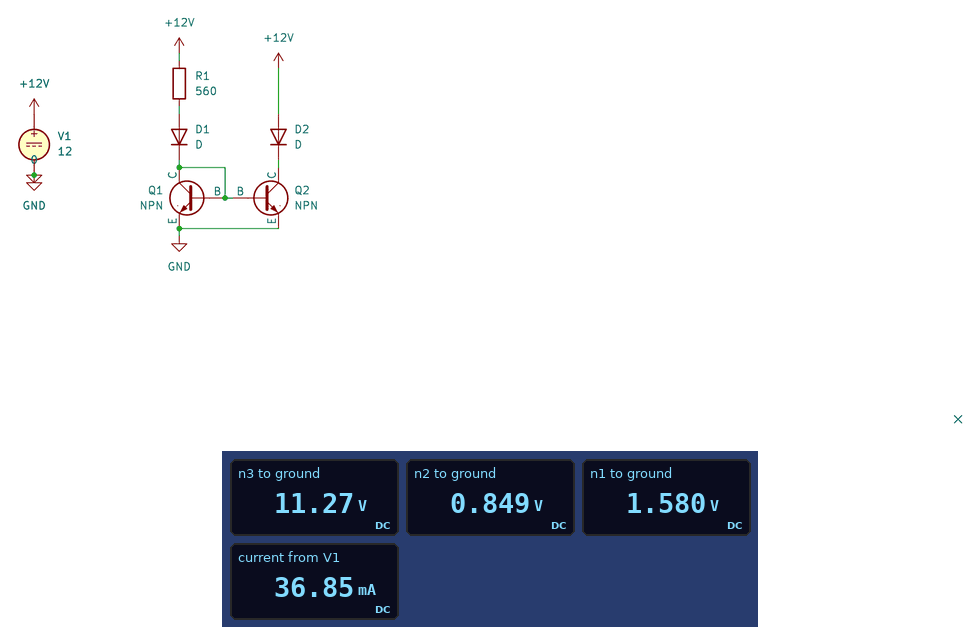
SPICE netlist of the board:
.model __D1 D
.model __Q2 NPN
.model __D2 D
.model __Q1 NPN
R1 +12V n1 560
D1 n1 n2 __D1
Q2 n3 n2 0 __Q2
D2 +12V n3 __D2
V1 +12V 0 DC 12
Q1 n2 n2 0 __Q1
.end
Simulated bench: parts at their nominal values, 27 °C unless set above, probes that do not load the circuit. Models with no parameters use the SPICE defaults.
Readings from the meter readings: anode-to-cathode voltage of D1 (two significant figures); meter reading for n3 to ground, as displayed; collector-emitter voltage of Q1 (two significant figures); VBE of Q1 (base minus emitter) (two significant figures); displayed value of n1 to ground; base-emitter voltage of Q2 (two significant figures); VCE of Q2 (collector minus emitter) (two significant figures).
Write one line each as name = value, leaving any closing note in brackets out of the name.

anode-to-cathode voltage of D1 = 730 mV
meter reading for n3 to ground, as displayed = 11.27 V
collector-emitter voltage of Q1 = 850 mV
VBE of Q1 (base minus emitter) = 850 mV
displayed value of n1 to ground = 1.580 V
base-emitter voltage of Q2 = 850 mV
VCE of Q2 (collector minus emitter) = 11 V
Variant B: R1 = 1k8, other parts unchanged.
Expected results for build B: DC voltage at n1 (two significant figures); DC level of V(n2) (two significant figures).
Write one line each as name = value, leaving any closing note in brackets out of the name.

DC voltage at n1 = 1.5 V
DC level of V(n2) = 820 mV
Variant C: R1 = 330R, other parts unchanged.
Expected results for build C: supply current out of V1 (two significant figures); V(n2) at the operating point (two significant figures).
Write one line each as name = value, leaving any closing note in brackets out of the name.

supply current out of V1 = 62 mA
V(n2) at the operating point = 860 mV
